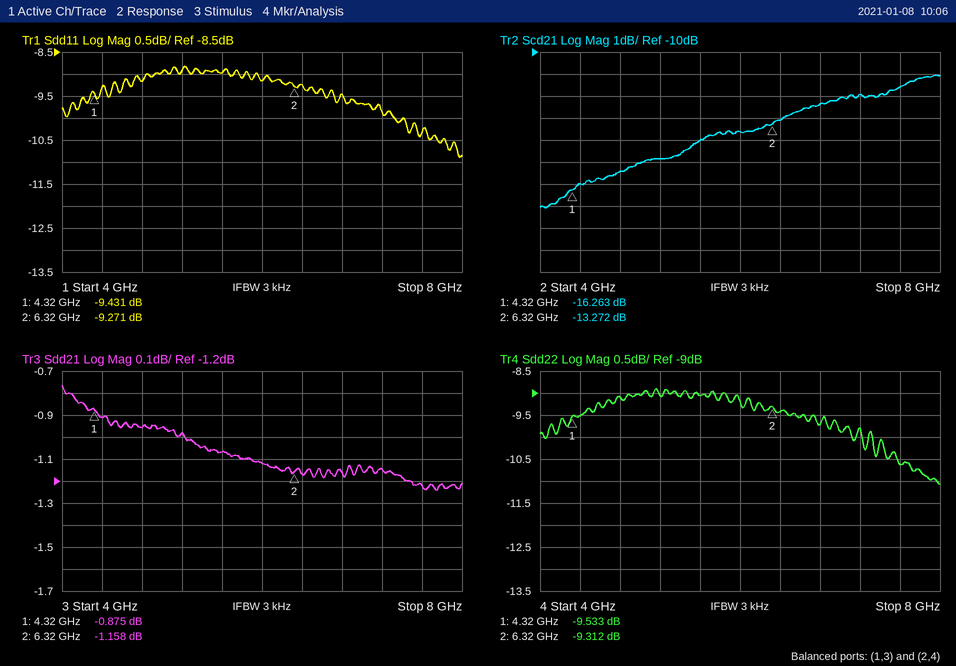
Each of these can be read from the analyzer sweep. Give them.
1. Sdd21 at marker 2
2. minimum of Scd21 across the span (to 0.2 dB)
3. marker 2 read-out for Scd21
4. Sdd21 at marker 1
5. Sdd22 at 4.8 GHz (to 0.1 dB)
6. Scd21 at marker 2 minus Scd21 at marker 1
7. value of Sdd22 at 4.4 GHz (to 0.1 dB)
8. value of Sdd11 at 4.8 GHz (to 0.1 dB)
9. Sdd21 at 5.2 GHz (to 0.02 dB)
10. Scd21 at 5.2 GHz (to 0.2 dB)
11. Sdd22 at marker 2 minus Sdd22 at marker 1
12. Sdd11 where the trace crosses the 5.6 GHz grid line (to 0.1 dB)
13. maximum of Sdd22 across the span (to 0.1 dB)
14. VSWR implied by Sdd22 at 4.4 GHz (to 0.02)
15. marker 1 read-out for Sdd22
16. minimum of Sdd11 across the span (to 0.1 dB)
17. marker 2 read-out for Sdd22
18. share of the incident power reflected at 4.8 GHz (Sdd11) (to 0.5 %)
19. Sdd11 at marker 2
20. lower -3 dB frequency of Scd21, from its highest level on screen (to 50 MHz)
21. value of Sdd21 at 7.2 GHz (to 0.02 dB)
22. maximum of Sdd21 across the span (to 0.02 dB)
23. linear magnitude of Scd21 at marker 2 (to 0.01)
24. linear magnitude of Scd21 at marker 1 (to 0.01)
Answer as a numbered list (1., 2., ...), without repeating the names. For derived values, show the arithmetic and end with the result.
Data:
1. -1.158 dB
2. -17.0 dB
3. -13.272 dB
4. -0.875 dB
5. -9.1 dB
6. -13.272 − (-16.263) = 2.991 dB
7. -9.5 dB
8. -9.2 dB
9. -0.98 dB
10. -14.8 dB
11. -9.312 − (-9.533) = 0.221 dB
12. -9.0 dB
13. -8.9 dB
14. |Γ| = 10^(-9.5/20) = 0.3350; VSWR = (1 + 0.3350)/(1 − 0.3350) ≈ 2.01, so 2.00 to the nearest 0.02
15. -9.533 dB
16. -10.9 dB
17. -9.312 dB
18. 10^(-9.2/10) ≈ 12.0 %
19. -9.271 dB
20. 5.60 GHz
21. -1.14 dB
22. -0.76 dB
23. 10^(-13.272/20) ≈ 0.22
24. 10^(-16.263/20) ≈ 0.15
